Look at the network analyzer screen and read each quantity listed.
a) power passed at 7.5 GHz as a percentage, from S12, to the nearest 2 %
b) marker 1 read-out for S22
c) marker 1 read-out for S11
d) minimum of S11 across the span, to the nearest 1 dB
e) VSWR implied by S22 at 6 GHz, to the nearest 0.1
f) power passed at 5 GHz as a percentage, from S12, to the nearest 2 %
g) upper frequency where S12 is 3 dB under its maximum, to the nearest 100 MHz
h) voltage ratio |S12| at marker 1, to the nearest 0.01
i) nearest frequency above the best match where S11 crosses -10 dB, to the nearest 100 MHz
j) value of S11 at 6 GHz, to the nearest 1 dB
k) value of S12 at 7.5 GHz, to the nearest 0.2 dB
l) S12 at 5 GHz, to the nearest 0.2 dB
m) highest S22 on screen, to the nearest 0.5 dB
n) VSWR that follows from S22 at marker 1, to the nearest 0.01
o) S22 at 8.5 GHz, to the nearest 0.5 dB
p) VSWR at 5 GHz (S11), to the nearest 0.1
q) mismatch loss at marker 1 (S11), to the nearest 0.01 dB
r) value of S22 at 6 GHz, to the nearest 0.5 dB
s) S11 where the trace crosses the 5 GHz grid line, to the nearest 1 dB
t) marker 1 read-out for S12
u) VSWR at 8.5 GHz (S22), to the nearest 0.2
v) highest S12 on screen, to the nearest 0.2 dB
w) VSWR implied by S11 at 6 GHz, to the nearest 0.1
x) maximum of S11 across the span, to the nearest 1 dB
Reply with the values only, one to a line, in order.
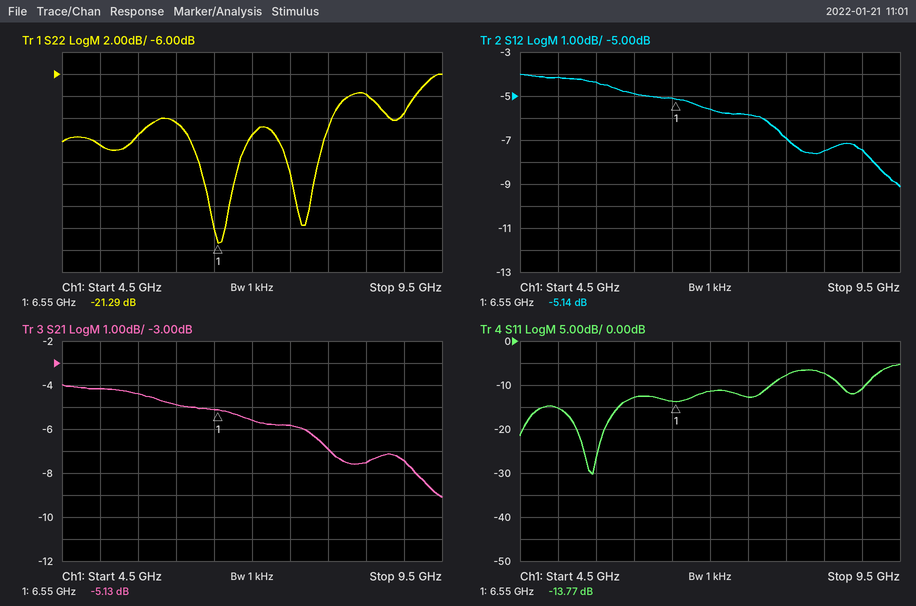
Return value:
26 %
-21.29 dB
-13.77 dB
-30 dB
1.9
38 %
8.0 GHz
0.55
7.8 GHz
-13 dB
-5.8 dB
-4.2 dB
-6.0 dB
1.19
-8.0 dB
1.4
0.19 dB
-10.5 dB
-15 dB
-5.14 dB
2.4
-4.0 dB
1.6
-5 dB
